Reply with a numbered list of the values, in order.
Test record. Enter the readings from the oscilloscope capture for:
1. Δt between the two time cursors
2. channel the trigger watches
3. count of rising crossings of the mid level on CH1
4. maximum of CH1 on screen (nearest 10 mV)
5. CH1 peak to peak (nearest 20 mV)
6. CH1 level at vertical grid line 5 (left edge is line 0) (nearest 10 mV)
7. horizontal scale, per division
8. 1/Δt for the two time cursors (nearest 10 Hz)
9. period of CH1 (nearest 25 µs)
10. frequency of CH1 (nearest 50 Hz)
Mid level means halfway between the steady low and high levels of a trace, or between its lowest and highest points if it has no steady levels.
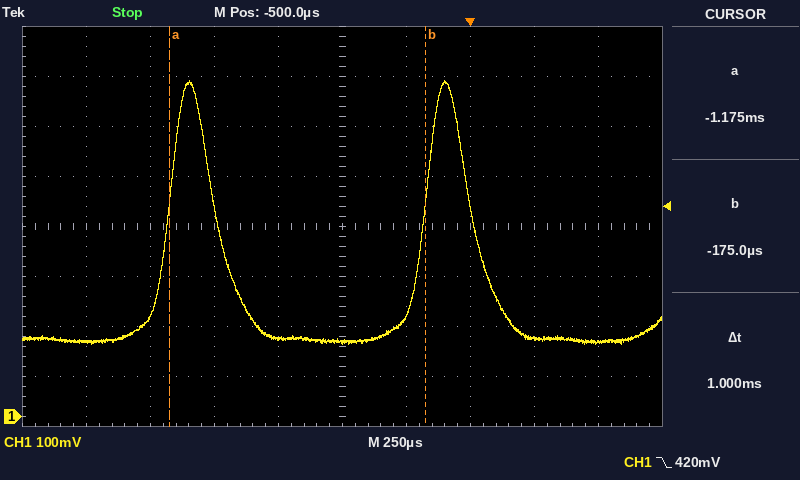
1. 1 ms
2. CH1
3. 2
4. 670 mV
5. 520 mV
6. 150 mV
7. 250 µs
8. 1.00 kHz
9. 1.000 ms
10. 1.00 kHz
